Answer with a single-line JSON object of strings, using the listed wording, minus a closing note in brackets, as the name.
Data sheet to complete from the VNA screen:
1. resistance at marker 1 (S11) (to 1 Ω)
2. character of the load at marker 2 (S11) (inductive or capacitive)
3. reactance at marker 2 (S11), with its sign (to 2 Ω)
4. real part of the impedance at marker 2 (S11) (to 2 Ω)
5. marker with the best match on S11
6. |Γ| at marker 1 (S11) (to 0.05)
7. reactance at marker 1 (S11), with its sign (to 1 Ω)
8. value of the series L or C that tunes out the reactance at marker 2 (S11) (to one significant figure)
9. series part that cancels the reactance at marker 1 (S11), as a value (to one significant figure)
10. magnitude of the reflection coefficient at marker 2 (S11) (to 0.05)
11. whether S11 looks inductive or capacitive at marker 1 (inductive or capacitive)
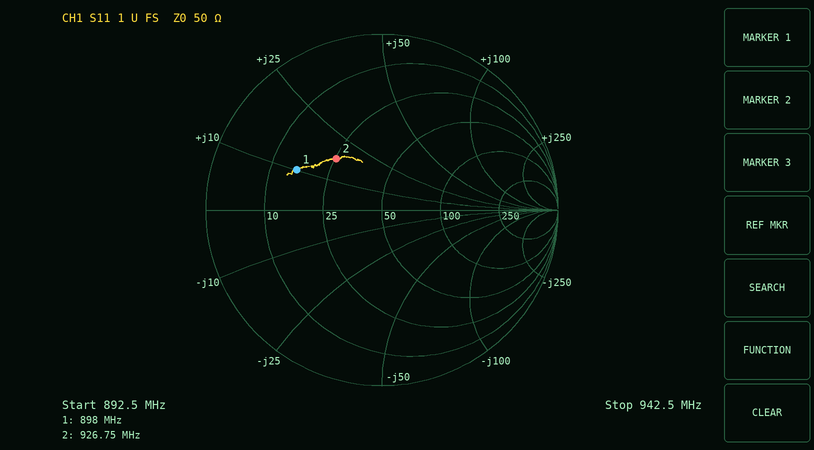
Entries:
{"resistance at marker 1 (S11)": "16 Ω", "character of the load at marker 2 (S11)": "inductive", "reactance at marker 2 (S11), with its sign": "+18 Ω", "real part of the impedance at marker 2 (S11)": "26 Ω", "marker with the best match on S11": "marker 2", "|Γ| at marker 1 (S11)": "0.55", "reactance at marker 1 (S11), with its sign": "+10 Ω", "value of the series L or C that tunes out the reactance at marker 2 (S11)": "10 pF", "series part that cancels the reactance at marker 1 (S11), as a value": "20 pF", "magnitude of the reflection coefficient at marker 2 (S11)": "0.40", "whether S11 looks inductive or capacitive at marker 1": "inductive"}
